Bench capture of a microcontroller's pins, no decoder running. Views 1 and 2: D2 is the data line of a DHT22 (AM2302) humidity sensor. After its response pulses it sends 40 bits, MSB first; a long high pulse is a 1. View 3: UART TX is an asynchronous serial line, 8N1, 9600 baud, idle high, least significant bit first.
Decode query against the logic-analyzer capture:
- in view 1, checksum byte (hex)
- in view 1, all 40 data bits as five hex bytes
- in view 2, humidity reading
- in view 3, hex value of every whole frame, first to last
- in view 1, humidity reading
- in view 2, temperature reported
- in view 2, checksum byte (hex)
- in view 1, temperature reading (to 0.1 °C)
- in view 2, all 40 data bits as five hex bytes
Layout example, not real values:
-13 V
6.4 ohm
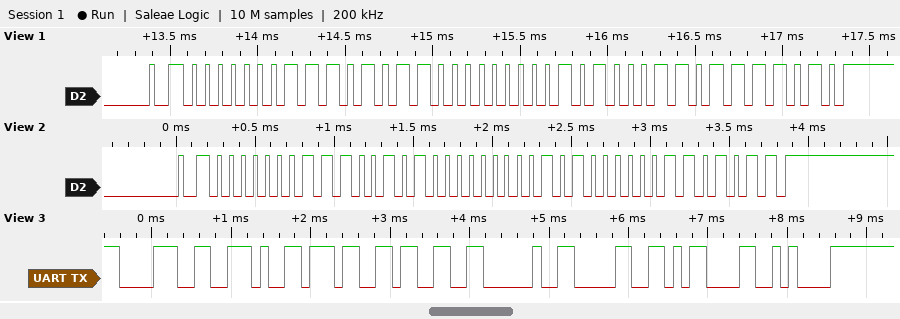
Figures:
0x7A
01 D6 00 A3 7A
45.8 %
0x38 0x2E 0x37 0x33 0x20 0x30 0x0D 0x0A
47.0 %
16.0 °C
0x6B
16.3 °C
01 CA 00 A0 6B
